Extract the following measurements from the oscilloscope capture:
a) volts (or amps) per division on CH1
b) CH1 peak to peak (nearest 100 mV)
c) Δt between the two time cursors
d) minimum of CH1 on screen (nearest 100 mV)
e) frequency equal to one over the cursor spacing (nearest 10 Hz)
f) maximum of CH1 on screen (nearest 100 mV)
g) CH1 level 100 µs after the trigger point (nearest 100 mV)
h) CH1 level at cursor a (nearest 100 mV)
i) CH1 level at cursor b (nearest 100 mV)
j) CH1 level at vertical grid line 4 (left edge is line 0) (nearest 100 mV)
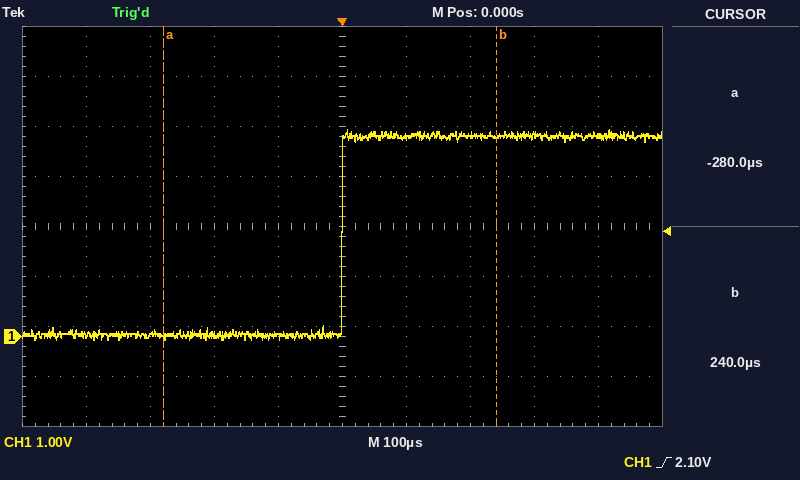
1 V
4.2 V
520 µs
-100 mV
1.92 kHz
4.1 V
4.0 V
0.0 V
4.0 V
0.0 V
